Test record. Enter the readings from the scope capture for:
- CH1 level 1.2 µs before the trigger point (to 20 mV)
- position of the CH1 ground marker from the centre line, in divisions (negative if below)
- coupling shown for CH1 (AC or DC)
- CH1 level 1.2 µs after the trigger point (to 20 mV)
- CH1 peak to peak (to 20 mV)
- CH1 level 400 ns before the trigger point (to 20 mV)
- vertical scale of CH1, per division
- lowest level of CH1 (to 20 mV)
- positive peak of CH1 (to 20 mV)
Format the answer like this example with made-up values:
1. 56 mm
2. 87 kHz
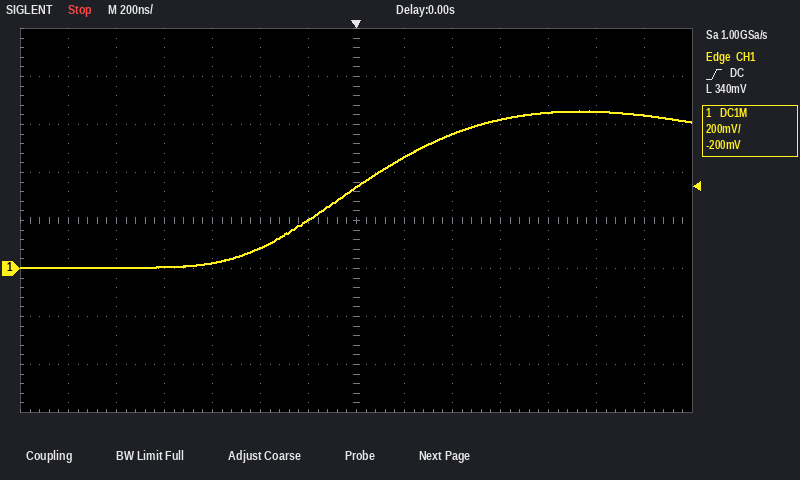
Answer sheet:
1. 0 mV
2. -1.0 div
3. DC
4. 640 mV
5. 660 mV
6. 80 mV
7. 200 mV
8. 0 mV
9. 660 mV
